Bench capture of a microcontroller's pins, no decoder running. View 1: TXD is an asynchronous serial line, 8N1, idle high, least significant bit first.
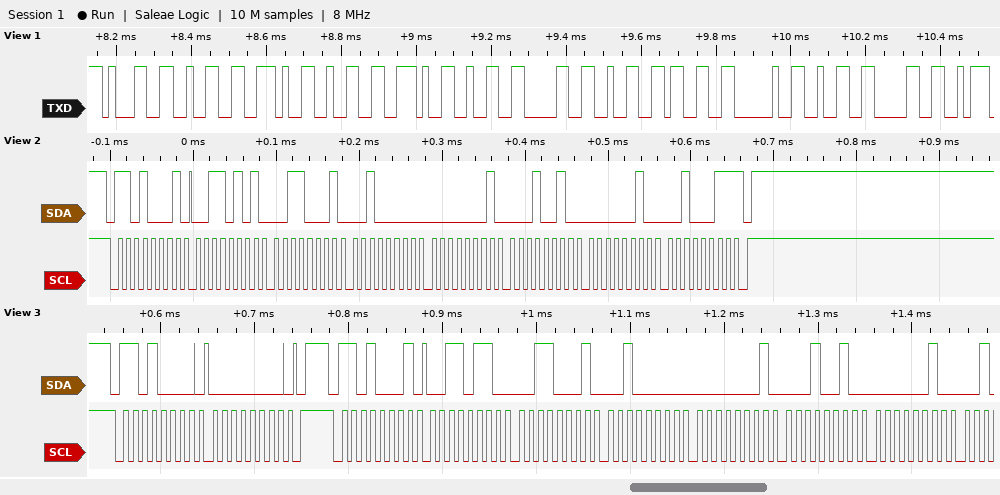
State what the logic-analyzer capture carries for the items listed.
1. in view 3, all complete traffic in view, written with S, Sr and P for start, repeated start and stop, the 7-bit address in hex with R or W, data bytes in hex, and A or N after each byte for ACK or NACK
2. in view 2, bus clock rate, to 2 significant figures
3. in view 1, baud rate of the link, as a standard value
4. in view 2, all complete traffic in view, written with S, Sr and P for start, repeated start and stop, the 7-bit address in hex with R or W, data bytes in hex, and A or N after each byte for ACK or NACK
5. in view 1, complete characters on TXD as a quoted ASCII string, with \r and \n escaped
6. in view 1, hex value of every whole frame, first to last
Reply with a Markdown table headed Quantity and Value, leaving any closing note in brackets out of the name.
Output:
| Quantity | Value |
|---|---|
| in view 3, all complete traffic in view, written with S, Sr and P for start, repeated start and stop, the 7-bit address in hex with R or W, data bytes in hex, and A or N after each byte for ACK or NACK | S 68W A 00 A P S 68R A 36 A 31 A 20 A 01 A 12 A 02 A |
| in view 2, bus clock rate, to 2 significant figures | 100 kHz |
| in view 1, baud rate of the link, as a standard value | 57600 baud |
| in view 2, all complete traffic in view, written with S, Sr and P for start, repeated start and stop, the 7-bit address in hex with R or W, data bytes in hex, and A or N after each byte for ACK or NACK | S 68R A 35 A 31 A 20 A 01 A 12 A 02 A 23 N P |
| in view 1, complete characters on TXD as a quoted ASCII string, with \r and \n escaped | "12.2.2023 20" |
| in view 1, hex value of every whole frame, first to last | 0x31 0x32 0x2E 0x32 0x2E 0x32 0x30 0x32 0x33 0x20 0x32 0x30 |
